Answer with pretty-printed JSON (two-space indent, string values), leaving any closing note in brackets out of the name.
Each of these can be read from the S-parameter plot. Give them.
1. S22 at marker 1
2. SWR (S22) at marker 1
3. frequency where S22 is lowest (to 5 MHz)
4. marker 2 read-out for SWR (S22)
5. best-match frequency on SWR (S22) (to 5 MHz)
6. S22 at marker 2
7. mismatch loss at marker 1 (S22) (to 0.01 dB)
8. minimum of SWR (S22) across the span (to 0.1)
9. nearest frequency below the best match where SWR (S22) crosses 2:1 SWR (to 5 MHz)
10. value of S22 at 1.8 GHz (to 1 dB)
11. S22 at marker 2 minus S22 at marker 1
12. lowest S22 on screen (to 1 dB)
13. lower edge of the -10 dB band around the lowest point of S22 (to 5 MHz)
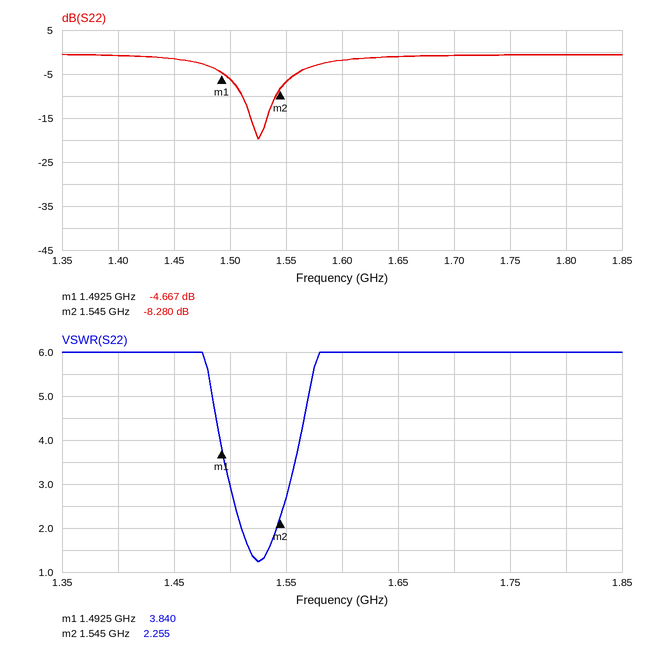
{
  "S22 at marker 1": "-4.667 dB",
  "SWR (S22) at marker 1": "3.840",
  "frequency where S22 is lowest": "1.525 GHz",
  "marker 2 read-out for SWR": "2.255",
  "best-match frequency on SWR (S22)": "1.525 GHz",
  "S22 at marker 2": "-8.280 dB",
  "mismatch loss at marker 1 (S22)": "1.81 dB",
  "minimum of SWR (S22) across the span": "1.2",
  "nearest frequency below the best match where SWR (S22) crosses 2:1 SWR": "1.510 GHz",
  "value of S22 at 1.8 GHz": "-1 dB",
  "S22 at marker 2 minus S22 at marker 1": "-3.613 dB",
  "lowest S22 on screen": "-20 dB",
  "lower edge of the -10 dB band around the lowest point of S22": "1.510 GHz"
}
